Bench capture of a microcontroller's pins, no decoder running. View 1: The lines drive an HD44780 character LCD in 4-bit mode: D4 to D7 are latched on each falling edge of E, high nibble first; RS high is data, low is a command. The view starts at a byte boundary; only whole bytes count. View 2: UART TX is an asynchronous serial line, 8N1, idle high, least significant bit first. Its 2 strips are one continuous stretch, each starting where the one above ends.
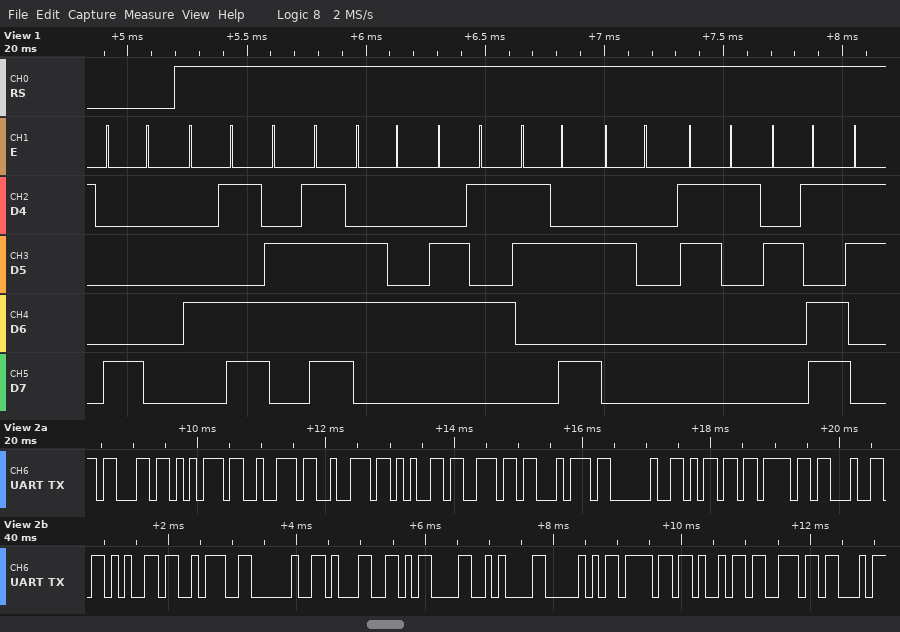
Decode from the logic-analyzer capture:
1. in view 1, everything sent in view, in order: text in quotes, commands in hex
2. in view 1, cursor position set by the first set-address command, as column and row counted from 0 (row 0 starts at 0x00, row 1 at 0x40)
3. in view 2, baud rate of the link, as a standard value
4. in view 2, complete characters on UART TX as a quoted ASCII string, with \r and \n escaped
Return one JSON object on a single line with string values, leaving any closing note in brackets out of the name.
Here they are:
{"in view 1, everything sent in view, in order: text in quotes, commands in hex": "0x80 \"Mode: 1-\"", "in view 1, cursor position set by the first set-address command, as column and row counted from 0": "column 0, row 0", "in view 2, baud rate of the link, as a standard value": "9600 baud", "in view 2, complete characters on UART TX as a quoted ASCII string, with \\r and \\n escaped": "\"current mode: 1\\r\\nPoin\""}
